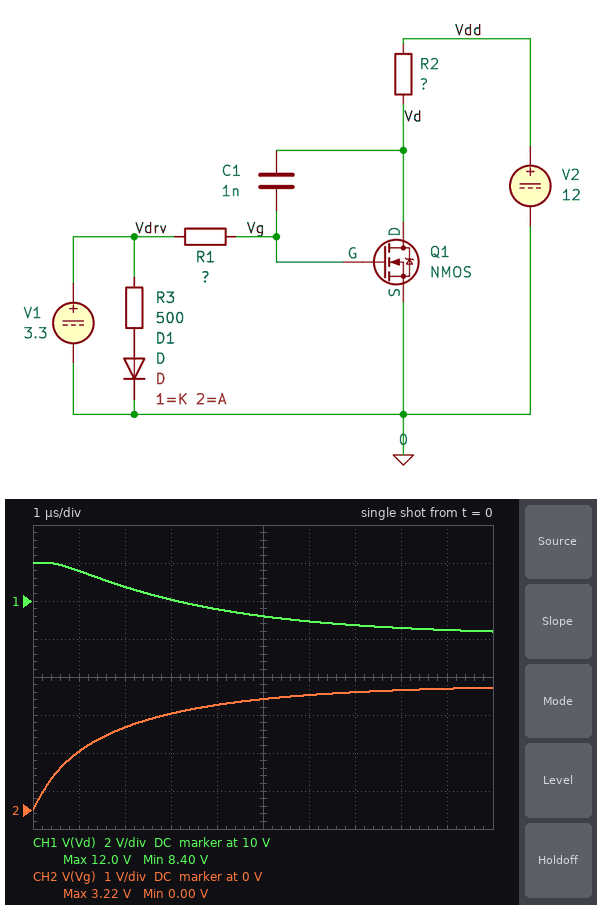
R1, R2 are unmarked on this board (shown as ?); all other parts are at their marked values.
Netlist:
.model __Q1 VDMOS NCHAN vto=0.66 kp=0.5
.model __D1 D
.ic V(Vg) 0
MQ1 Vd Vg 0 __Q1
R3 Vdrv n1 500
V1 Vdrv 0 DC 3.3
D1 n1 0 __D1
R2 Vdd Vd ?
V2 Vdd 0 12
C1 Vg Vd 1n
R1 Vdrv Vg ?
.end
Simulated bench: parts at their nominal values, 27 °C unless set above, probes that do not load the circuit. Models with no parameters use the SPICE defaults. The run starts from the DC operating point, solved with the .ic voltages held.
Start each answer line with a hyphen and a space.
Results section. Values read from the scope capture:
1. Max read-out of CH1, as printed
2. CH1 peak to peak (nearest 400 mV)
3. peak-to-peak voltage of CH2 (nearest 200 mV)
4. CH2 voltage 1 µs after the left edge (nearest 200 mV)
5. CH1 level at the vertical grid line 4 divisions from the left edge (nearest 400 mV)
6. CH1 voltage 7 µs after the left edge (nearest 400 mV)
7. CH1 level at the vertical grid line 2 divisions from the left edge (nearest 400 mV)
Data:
- 12.0 V
- 3.6 V
- 3.2 V
- 1.6 V
- 9.6 V
- 8.8 V
- 10.8 V
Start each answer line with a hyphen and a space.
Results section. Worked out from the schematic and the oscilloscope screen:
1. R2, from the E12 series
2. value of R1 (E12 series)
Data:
- 2.2 Ω
- 560 Ω
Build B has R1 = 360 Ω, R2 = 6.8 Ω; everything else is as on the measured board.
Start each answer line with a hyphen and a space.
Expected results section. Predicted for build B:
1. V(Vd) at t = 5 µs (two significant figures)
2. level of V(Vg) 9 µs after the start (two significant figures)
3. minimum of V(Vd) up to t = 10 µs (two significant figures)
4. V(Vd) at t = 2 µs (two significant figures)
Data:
- 4.3 V
- 3.0 V
- 2.3 V
- 8.1 V
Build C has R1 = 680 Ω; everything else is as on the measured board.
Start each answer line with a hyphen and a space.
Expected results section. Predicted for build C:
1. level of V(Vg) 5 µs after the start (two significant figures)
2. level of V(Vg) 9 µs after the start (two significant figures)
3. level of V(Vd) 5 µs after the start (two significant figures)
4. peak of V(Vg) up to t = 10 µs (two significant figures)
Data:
- 2.8 V
- 3.1 V
- 9.5 V
- 3.2 V
